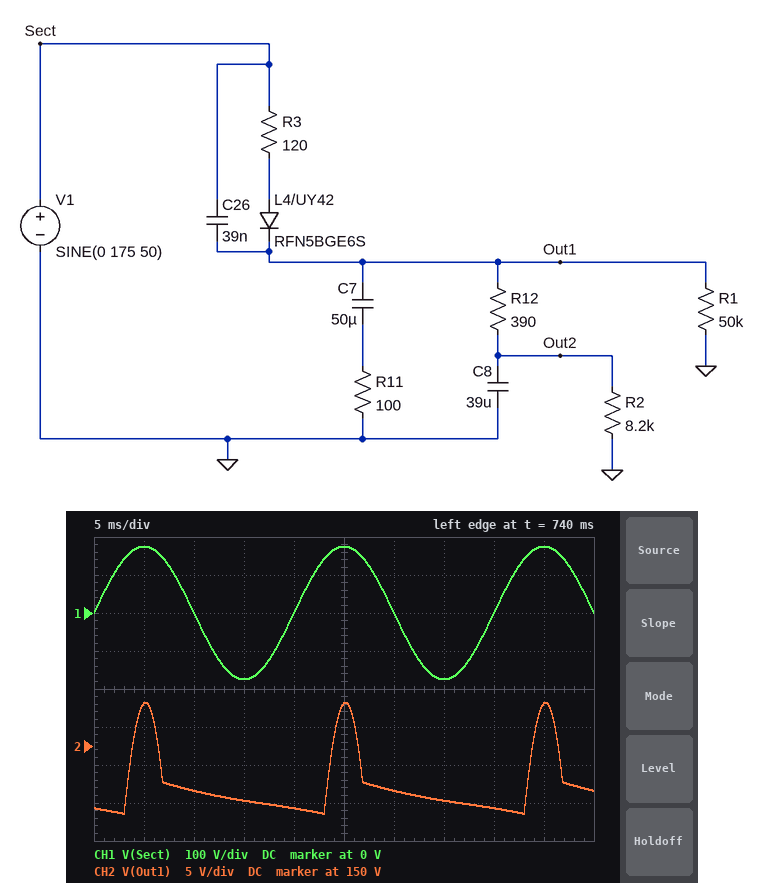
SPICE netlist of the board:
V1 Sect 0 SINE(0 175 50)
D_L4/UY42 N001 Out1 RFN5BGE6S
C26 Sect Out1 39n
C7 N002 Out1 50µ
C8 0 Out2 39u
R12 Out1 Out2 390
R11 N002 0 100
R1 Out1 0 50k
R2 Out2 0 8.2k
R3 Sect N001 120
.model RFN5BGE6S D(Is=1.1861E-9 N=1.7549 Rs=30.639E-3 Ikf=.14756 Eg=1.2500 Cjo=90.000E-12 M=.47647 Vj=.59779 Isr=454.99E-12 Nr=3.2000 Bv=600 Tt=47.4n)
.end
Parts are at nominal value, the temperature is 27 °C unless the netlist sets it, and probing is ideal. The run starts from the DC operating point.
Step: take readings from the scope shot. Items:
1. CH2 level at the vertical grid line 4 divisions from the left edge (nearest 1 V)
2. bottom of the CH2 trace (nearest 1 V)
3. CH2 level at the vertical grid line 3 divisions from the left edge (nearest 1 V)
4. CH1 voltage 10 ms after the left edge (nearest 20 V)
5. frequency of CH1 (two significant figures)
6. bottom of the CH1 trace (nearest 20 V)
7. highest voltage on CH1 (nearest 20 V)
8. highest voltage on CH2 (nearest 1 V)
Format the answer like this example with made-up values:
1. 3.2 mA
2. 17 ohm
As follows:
1. 142 V
2. 141 V
3. 143 V
4. 0 V
5. 50 Hz
6. -180 V
7. 180 V
8. 156 V
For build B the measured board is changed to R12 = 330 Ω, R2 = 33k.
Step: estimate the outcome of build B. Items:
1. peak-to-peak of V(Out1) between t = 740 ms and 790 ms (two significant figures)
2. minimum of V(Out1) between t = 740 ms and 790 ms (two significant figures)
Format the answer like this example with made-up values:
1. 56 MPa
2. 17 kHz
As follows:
1. 7.4 V
2. 160 V
